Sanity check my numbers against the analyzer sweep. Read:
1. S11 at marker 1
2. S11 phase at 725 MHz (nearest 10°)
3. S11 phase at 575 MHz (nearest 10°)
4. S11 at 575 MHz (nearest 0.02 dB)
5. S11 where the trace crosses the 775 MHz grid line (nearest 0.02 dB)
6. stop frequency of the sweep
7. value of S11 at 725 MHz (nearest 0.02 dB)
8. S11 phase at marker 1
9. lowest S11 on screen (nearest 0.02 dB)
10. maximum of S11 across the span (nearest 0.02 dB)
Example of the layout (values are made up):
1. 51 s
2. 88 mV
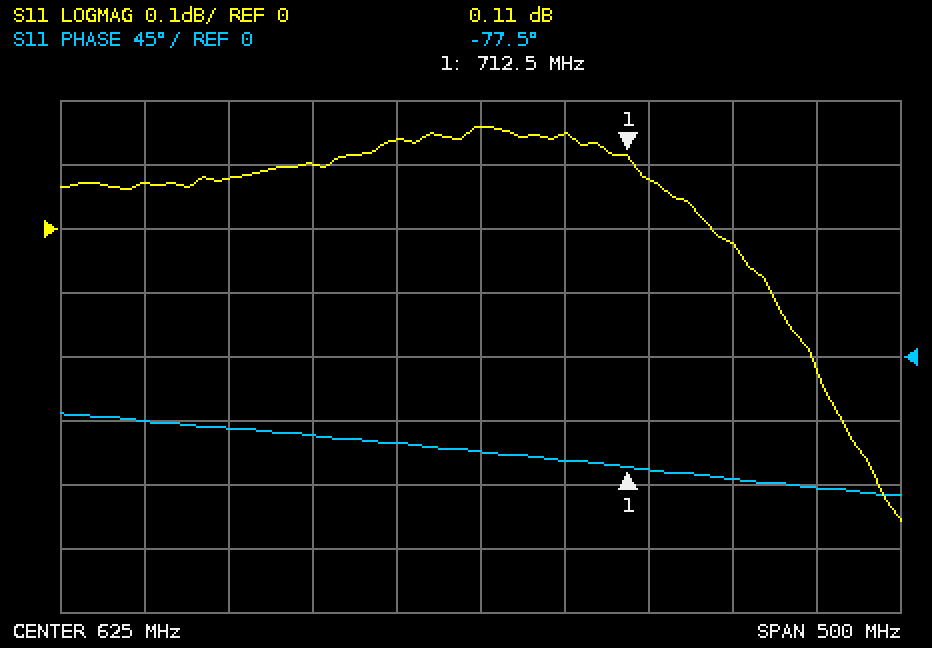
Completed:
1. 0.11 dB
2. -80°
3. -60°
4. 0.14 dB
5. -0.02 dB
6. 875 MHz
7. 0.08 dB
8. -77.5°
9. -0.46 dB
10. 0.16 dB
